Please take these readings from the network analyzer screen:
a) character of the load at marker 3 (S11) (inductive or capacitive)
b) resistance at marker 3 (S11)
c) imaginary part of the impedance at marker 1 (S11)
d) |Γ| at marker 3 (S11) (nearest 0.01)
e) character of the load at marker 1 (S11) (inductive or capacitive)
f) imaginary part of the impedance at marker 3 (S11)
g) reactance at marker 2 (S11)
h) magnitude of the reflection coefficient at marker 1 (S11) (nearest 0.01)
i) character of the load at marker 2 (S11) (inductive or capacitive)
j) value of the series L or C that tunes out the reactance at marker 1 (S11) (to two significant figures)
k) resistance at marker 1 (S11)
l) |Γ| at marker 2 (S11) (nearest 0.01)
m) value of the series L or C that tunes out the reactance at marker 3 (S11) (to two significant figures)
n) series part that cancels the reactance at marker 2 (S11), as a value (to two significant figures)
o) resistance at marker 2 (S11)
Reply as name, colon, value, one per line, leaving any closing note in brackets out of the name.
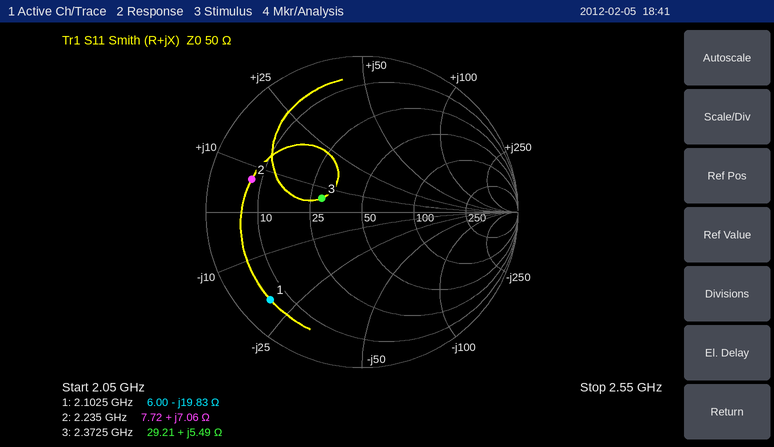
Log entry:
character of the load at marker 3 (S11): inductive
resistance at marker 3: 29.21 Ω
imaginary part of the impedance at marker 1: -19.83 Ω
|Γ| at marker 3 (S11): 0.27
character of the load at marker 1 (S11): capacitive
imaginary part of the impedance at marker 3: +5.49 Ω
reactance at marker 2: +7.06 Ω
magnitude of the reflection coefficient at marker 1 (S11): 0.81
character of the load at marker 2 (S11): inductive
value of the series L or C that tunes out the reactance at marker 1 (S11): 1.5 nH
resistance at marker 1: 6.00 Ω
|Γ| at marker 2 (S11): 0.74
value of the series L or C that tunes out the reactance at marker 3 (S11): 12 pF
series part that cancels the reactance at marker 2 (S11), as a value: 10 pF
resistance at marker 2: 7.72 Ω
